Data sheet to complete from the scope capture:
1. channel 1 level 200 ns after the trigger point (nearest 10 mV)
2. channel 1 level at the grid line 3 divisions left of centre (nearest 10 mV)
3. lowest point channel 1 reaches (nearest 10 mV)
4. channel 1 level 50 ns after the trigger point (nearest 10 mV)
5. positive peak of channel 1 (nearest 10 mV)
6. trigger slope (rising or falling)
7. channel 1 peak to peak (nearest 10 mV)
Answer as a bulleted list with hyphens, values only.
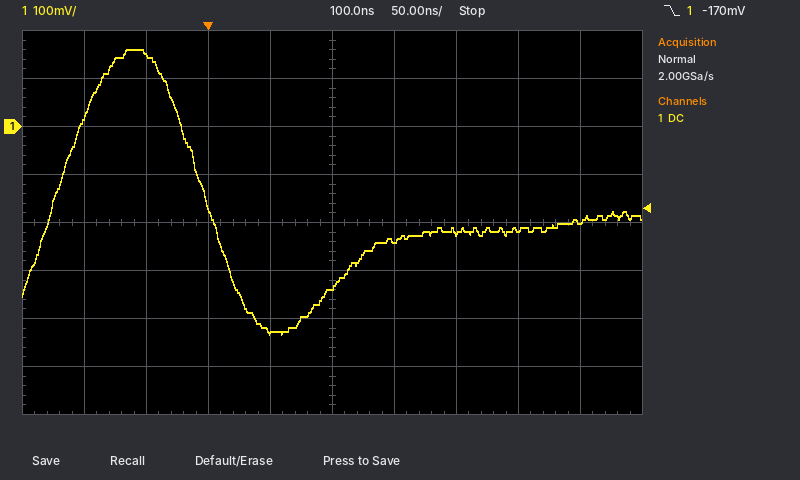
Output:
- -220 mV
- 150 mV
- -430 mV
- -430 mV
- 160 mV
- falling
- 590 mV
